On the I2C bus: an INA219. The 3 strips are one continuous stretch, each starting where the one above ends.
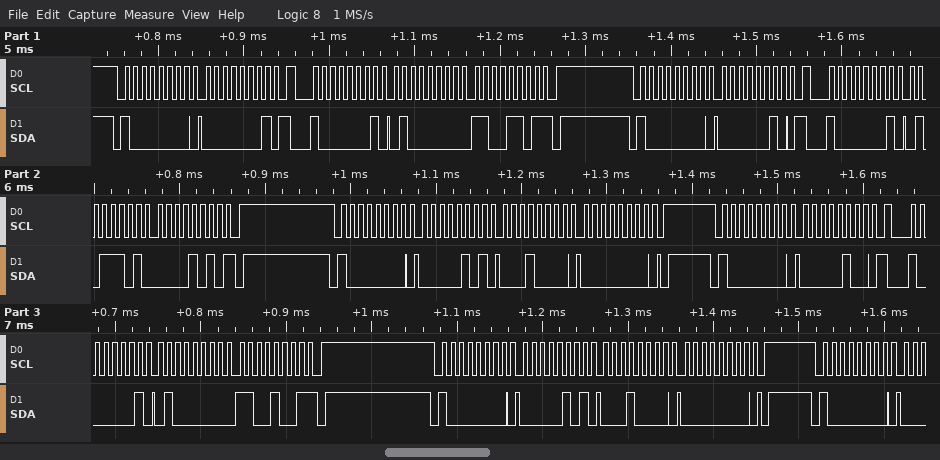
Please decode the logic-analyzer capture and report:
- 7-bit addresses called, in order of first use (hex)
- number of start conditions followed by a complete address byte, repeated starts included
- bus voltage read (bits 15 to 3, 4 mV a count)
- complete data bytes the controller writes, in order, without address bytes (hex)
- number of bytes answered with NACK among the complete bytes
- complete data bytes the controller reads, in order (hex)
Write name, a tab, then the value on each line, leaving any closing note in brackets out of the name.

7-bit addresses called, in order of first use	0x40
number of start conditions followed by a complete address byte, repeated starts included	9
bus voltage read	11.908 V
complete data bytes the controller writes, in order, without address bytes	01 02 05 10 00 04 05 10 00
number of bytes answered with NACK among the complete bytes	3
complete data bytes the controller reads, in order	40 CD 5D 0A 40 C9
